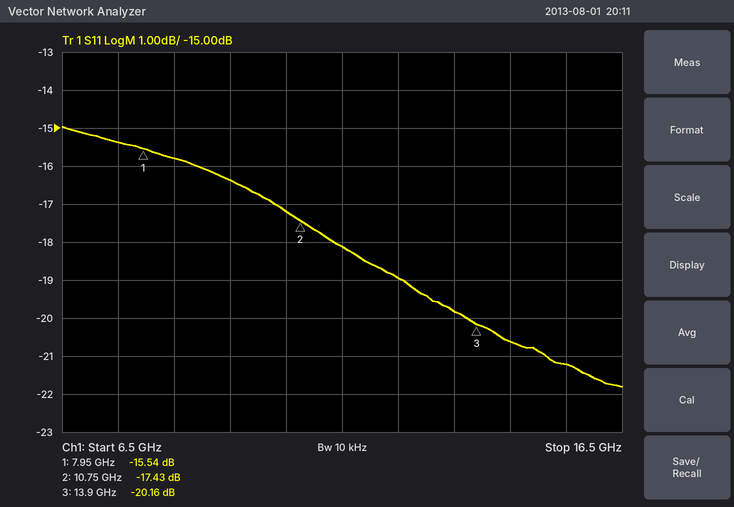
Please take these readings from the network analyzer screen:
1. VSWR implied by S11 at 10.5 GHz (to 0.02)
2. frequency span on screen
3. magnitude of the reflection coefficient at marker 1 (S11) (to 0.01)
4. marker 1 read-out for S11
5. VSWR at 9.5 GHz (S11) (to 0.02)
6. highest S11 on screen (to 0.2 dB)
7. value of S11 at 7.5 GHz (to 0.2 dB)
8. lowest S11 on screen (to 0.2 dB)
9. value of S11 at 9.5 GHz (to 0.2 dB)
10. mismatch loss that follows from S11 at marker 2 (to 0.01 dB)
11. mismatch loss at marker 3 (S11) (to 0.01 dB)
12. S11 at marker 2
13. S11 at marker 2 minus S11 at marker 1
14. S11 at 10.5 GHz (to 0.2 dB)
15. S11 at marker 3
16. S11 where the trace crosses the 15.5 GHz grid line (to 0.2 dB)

1.32
10 GHz
0.17
-15.54 dB
1.36
-15.0 dB
-15.4 dB
-21.8 dB
-16.4 dB
0.08 dB
0.04 dB
-17.43 dB
-1.89 dB
-17.2 dB
-20.16 dB
-21.2 dB
